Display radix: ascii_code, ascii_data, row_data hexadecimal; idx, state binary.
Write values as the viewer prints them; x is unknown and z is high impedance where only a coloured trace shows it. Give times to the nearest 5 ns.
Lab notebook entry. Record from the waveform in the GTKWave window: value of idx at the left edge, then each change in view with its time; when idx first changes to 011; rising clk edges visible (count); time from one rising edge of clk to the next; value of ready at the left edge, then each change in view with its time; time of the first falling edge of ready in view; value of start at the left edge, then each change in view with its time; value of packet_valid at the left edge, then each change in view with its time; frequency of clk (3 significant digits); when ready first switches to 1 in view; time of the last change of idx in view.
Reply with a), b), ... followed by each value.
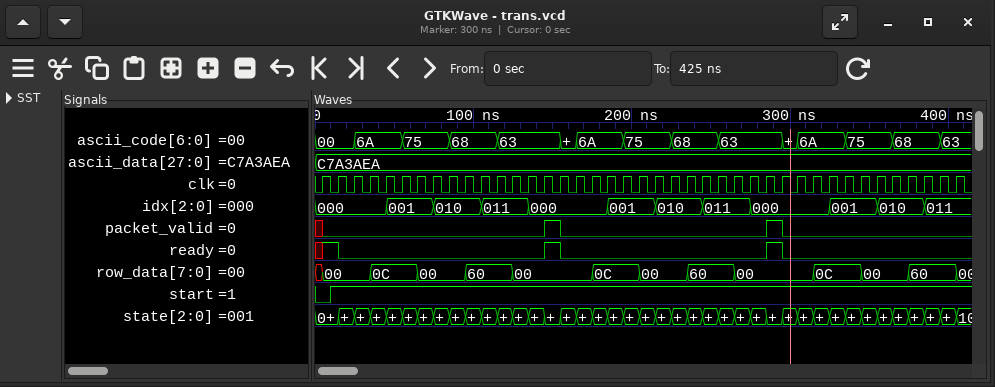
a) 000, 001 at 45 ns, 010 at 75 ns, 011 at 105 ns, 000 at 135 ns, 001 at 185 ns, 010 at 215 ns, 011 at 245 ns, 000 at 275 ns, 001 at 325 ns, 010 at 355 ns, 011 at 385 ns
b) 105 ns
c) 41
d) 10 ns
e) x, 1 at 5 ns, 0 at 15 ns, 1 at 145 ns, 0 at 155 ns, 1 at 285 ns, 0 at 295 ns
f) 15 ns
g) 0, 1 at 10 ns
h) x, 0 at 5 ns, 1 at 145 ns, 0 at 155 ns, 1 at 285 ns, 0 at 295 ns
i) 100 MHz
j) 5 ns
k) 385 ns
